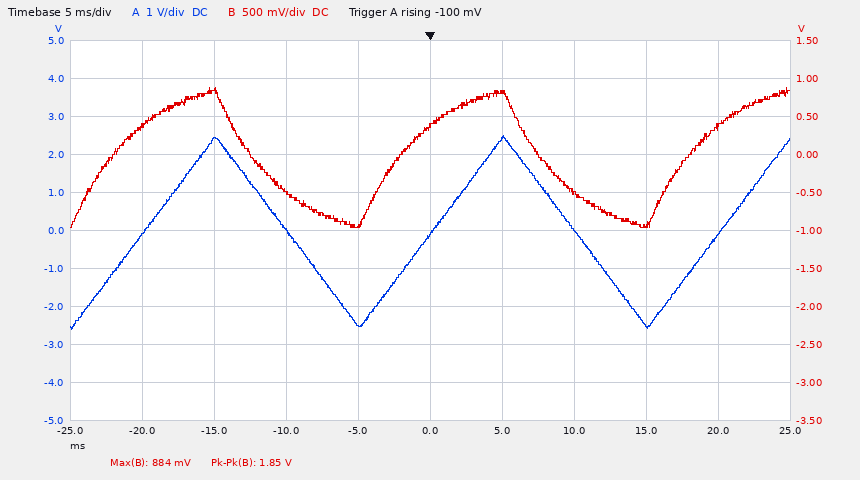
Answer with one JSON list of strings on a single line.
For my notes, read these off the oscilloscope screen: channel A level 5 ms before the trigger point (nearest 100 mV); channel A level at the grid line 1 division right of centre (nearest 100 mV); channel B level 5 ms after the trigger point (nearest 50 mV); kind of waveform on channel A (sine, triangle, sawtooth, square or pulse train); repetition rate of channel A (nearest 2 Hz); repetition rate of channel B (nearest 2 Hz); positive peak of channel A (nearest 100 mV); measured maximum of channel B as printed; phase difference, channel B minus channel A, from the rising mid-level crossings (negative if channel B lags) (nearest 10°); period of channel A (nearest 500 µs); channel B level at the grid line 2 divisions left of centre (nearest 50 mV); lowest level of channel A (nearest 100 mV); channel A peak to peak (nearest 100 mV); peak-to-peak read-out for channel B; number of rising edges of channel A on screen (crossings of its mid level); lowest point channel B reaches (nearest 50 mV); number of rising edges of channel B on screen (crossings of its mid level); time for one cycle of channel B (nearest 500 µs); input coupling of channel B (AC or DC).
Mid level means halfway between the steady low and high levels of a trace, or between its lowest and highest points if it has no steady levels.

["-2.5 V", "2.4 V", "800 mV", "triangle", "50 Hz", "50 Hz", "2.5 V", "884 mV", "+40°", "20.0 ms", "-500 mV", "-2.6 V", "5.1 V", "1.85 V", "3", "-950 mV", "3", "20.0 ms", "DC"]
